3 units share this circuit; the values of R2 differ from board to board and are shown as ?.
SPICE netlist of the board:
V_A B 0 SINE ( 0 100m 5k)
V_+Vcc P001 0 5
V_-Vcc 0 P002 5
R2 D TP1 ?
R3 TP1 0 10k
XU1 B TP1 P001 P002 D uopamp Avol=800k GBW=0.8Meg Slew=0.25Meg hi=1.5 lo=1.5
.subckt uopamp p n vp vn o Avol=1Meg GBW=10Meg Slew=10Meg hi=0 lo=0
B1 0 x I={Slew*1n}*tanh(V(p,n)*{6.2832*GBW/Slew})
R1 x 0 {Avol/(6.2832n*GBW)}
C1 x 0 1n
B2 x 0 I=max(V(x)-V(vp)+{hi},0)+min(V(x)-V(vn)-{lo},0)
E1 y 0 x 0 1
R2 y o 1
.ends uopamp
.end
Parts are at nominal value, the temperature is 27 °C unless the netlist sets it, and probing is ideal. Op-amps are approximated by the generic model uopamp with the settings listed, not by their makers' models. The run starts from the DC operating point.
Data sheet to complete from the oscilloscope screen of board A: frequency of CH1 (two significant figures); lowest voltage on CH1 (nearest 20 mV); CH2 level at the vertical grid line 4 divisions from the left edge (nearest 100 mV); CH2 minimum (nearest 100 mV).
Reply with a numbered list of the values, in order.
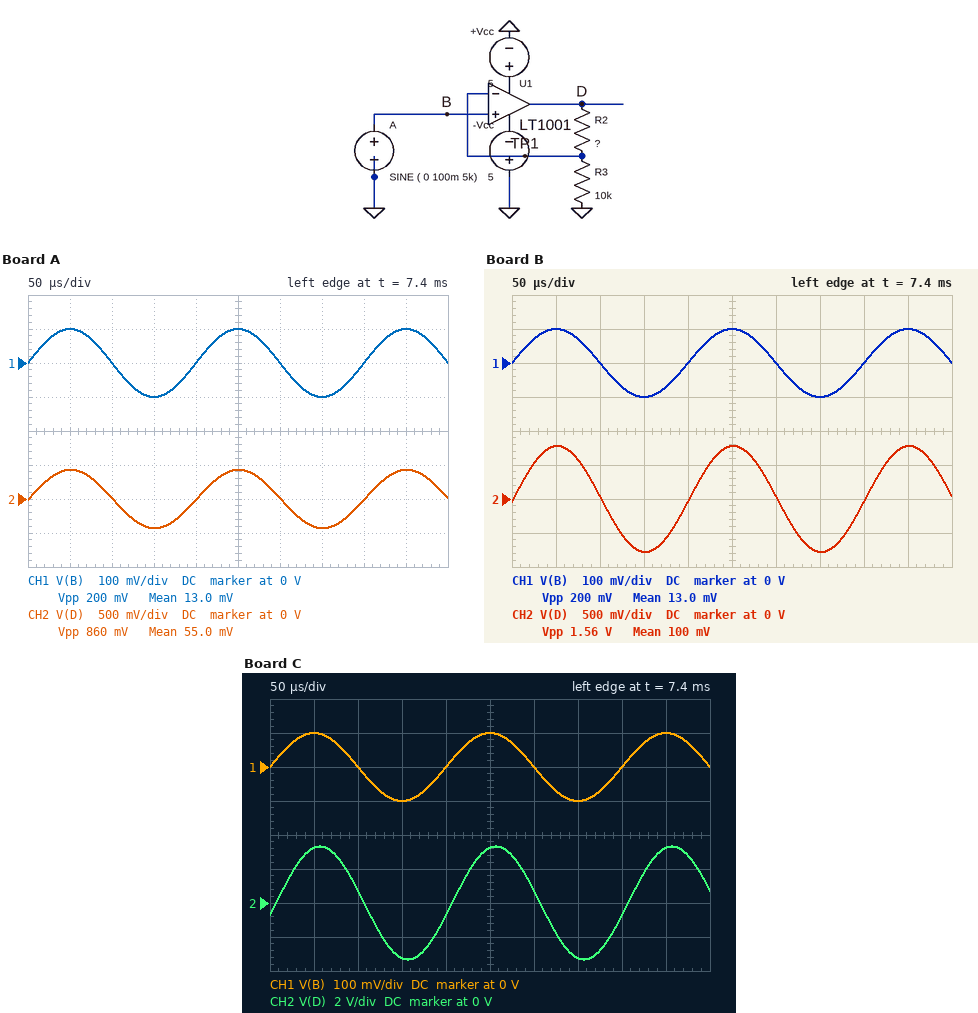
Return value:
1. 5.0 kHz
2. -100 mV
3. 0 V
4. -400 mV
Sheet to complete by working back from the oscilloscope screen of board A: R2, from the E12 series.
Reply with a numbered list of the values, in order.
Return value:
1. 33 kΩ
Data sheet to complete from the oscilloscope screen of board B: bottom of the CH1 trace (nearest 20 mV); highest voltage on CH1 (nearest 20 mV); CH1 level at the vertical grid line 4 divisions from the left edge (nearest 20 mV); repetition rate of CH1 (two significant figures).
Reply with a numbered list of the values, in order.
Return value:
1. -100 mV
2. 100 mV
3. 0 V
4. 5.0 kHz
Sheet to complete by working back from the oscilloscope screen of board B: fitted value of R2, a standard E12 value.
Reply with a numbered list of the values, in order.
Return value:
1. 68 kΩ
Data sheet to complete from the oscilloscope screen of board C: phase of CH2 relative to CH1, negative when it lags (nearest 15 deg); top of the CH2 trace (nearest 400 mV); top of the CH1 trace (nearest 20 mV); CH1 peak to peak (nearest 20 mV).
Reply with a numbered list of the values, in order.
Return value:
1. -15 deg
2. 3.2 V
3. 100 mV
4. 200 mV
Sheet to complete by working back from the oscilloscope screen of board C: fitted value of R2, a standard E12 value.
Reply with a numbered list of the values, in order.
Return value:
1. 330 kΩ
